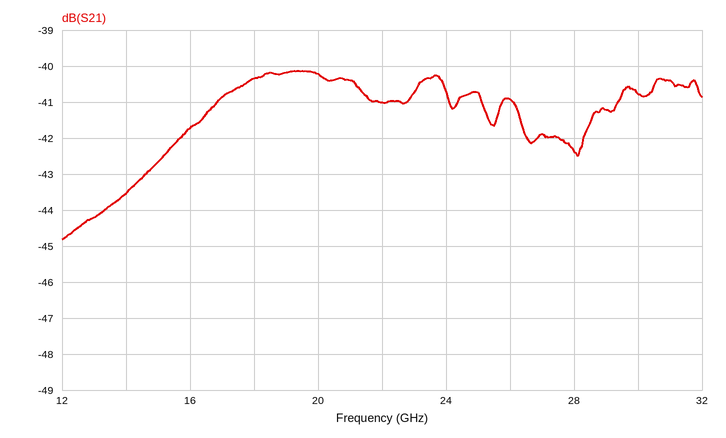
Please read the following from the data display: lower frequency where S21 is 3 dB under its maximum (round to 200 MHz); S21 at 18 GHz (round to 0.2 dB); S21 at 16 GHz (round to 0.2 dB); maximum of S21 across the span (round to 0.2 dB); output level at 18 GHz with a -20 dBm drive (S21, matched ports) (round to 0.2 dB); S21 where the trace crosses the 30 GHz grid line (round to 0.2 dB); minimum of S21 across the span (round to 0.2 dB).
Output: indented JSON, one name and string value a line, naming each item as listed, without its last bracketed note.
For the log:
{
  "lower frequency where S21 is 3 dB under its maximum": "14.4 GHz",
  "S21 at 18 GHz": "-40.4 dB",
  "S21 at 16 GHz": "-41.8 dB",
  "maximum of S21 across the span": "-40.2 dB",
  "output level at 18 GHz with a -20 dBm drive (S21, matched ports)": "-60.4 dBm",
  "S21 where the trace crosses the 30 GHz grid line": "-40.8 dB",
  "minimum of S21 across the span": "-44.8 dB"
}
